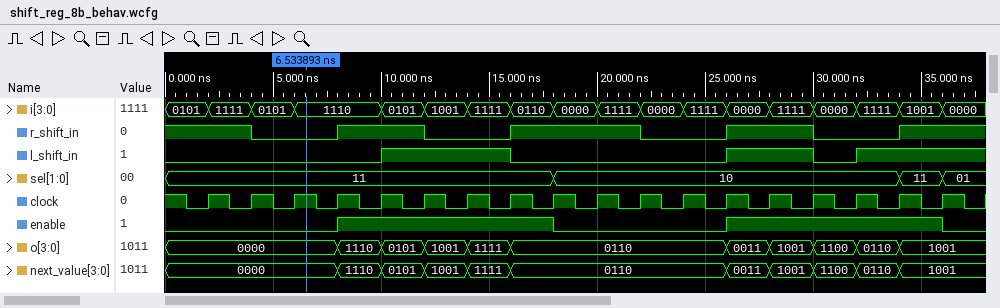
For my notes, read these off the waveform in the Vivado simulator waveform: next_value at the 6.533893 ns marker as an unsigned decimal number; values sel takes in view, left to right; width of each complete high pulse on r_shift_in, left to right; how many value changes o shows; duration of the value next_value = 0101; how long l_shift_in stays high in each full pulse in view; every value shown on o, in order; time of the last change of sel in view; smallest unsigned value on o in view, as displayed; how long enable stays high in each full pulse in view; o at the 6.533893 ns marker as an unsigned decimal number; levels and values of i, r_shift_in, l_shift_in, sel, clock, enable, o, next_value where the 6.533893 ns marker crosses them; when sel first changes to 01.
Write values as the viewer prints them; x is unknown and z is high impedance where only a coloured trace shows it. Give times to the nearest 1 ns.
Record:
0
11, 10, 11, 01
4 ns, 6 ns, 4 ns
10
2 ns
6 ns, 4 ns
0000, 1110, 0101, 1001, 1111, 0110, 0011, 1001, 1100, 0110, 1001
36 ns
0000
10 ns, 10 ns
0
i=1110, r_shift_in=0, l_shift_in=0, sel=11, clock=1, enable=0, o=0000, next_value=0000
36 ns
